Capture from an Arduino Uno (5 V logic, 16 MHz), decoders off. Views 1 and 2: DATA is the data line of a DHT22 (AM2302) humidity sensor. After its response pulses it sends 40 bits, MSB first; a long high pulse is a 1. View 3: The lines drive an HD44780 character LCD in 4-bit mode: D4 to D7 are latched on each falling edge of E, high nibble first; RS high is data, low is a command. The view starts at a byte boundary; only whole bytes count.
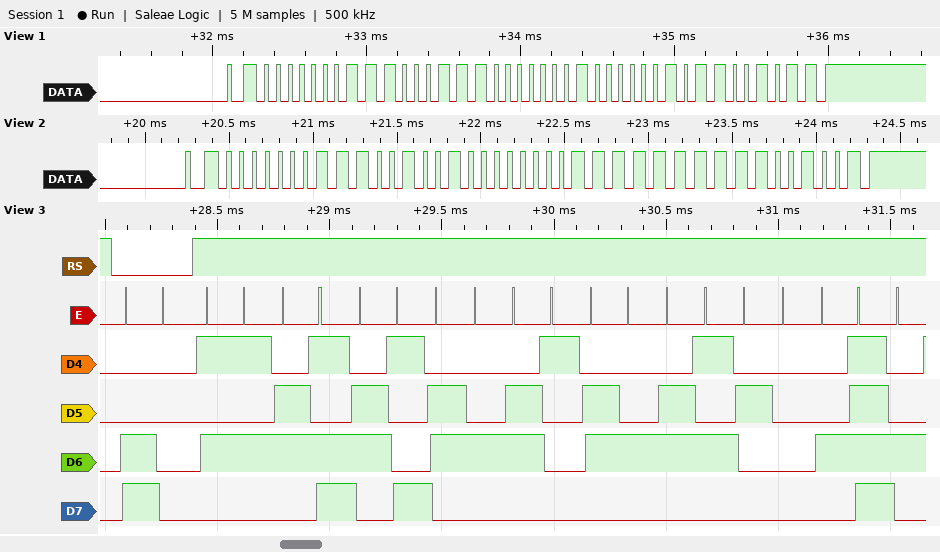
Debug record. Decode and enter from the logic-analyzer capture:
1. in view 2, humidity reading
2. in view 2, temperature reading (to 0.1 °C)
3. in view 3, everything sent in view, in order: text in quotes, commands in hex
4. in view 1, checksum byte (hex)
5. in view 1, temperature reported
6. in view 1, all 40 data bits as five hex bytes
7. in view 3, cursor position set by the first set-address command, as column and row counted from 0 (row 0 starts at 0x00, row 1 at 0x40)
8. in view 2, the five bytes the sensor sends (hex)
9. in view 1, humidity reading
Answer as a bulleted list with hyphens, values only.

- 45.7 %
- 25.5 °C
- 0xC0 "Umidade O"
- 0xCB
- 25.8 °C
- 01 C7 01 02 CB
- column 0, row 1
- 01 C9 00 FF C9
- 45.5 %
